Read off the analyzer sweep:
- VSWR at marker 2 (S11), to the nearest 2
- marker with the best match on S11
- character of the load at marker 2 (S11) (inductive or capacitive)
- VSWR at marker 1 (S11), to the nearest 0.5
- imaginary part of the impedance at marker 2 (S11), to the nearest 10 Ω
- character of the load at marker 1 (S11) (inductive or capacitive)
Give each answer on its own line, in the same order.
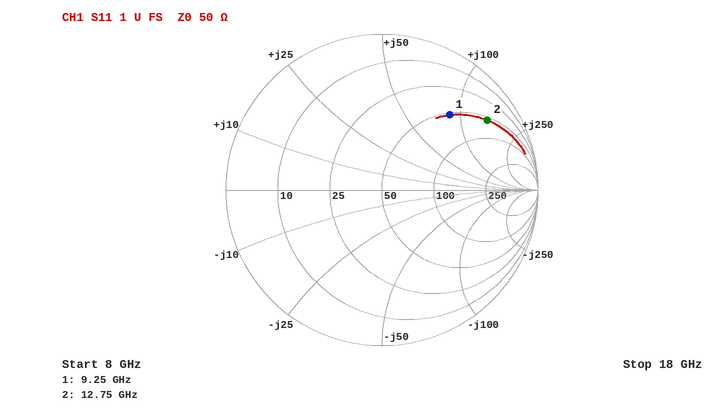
10
marker 1
inductive
4.5
+150 Ω
inductive
